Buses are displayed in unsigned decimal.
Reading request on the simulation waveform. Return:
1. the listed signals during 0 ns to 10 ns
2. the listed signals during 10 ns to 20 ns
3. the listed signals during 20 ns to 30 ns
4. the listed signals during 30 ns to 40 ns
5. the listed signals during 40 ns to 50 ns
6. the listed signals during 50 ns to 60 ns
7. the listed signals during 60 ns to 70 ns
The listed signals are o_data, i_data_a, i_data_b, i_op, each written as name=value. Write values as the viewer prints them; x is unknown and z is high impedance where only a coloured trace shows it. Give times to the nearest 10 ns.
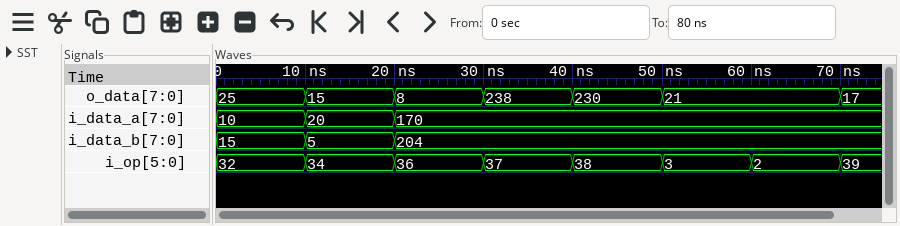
o_data=25, i_data_a=10, i_data_b=15, i_op=32
o_data=15, i_data_a=20, i_data_b=5, i_op=34
o_data=8, i_data_a=170, i_data_b=204, i_op=36
o_data=238, i_data_a=170, i_data_b=204, i_op=37
o_data=230, i_data_a=170, i_data_b=204, i_op=38
o_data=21, i_data_a=170, i_data_b=204, i_op=3
o_data=21, i_data_a=170, i_data_b=204, i_op=2
